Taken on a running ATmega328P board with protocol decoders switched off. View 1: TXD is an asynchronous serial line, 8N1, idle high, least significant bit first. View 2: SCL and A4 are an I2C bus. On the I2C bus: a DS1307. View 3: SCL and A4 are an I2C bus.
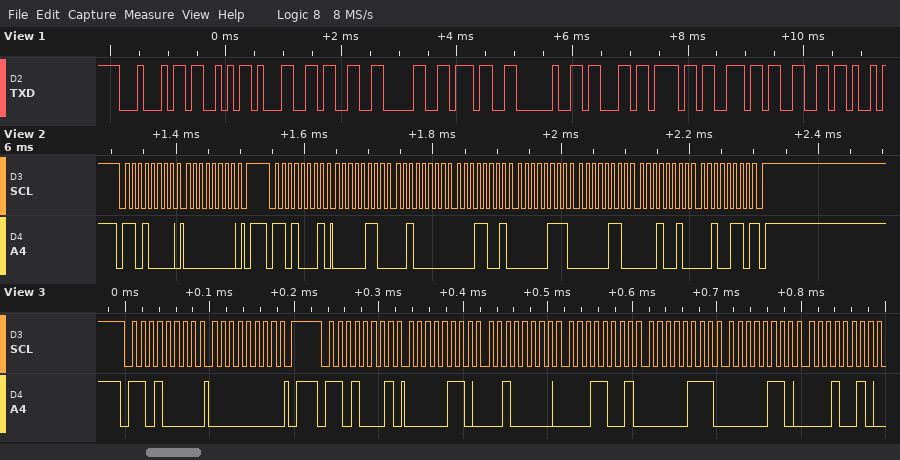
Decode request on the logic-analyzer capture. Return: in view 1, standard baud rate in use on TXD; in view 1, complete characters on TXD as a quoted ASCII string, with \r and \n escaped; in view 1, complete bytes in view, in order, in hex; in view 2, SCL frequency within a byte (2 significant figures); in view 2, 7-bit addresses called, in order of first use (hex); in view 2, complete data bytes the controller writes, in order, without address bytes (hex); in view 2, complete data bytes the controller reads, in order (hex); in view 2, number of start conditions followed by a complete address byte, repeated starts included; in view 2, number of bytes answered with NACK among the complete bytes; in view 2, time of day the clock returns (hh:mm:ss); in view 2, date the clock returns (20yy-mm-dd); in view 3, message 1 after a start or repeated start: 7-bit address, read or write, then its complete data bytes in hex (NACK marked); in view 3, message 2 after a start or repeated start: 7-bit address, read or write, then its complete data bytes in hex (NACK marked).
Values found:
9600 baud
"DS1307 conf"
0x44 0x53 0x31 0x33 0x30 0x37 0x20 0x63 0x6F 0x6E 0x66
100 kHz
0x68
00
06 20 19 07 06 12 26
2
1
19:20:06
2026-12-06
0x68 write: 00
0x68 read: 06 20 19 07 06 12
